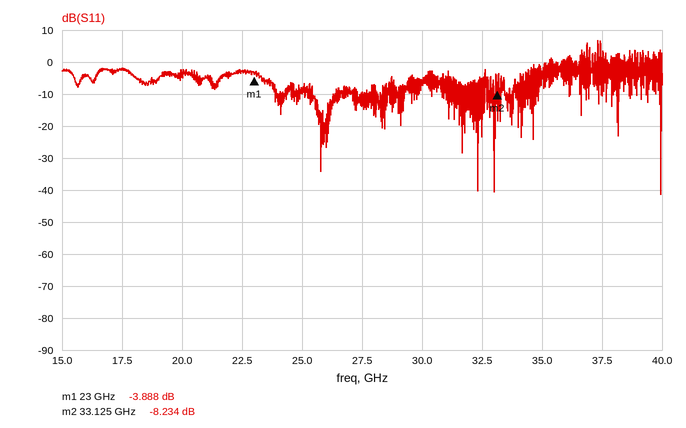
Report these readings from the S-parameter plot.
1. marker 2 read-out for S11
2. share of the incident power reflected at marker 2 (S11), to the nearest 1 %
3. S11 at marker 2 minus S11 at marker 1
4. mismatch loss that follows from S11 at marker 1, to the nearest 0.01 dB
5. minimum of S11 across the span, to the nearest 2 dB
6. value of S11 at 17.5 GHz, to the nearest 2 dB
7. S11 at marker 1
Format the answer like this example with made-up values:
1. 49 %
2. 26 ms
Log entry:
1. -8.234 dB
2. 15 %
3. -4.346 dB
4. 2.28 dB
5. -42 dB
6. -2 dB
7. -3.888 dB
